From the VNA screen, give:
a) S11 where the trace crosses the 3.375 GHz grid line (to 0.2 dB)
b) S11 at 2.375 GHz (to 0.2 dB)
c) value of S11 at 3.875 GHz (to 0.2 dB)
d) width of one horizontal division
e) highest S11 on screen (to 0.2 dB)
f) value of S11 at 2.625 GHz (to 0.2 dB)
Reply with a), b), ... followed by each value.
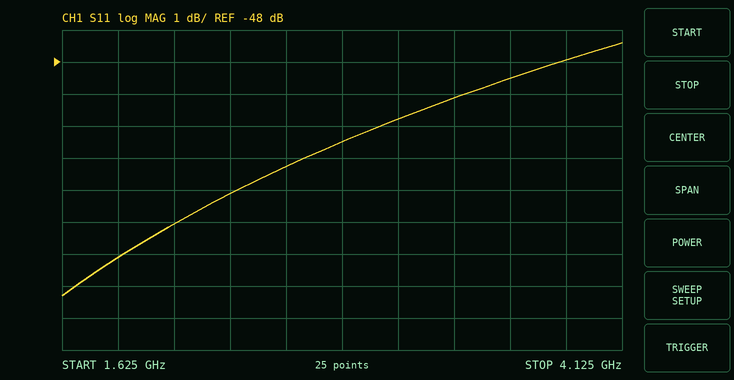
a) -49.2 dB
b) -52.2 dB
c) -48.0 dB
d) 250 MHz
e) -47.4 dB
f) -51.2 dB
